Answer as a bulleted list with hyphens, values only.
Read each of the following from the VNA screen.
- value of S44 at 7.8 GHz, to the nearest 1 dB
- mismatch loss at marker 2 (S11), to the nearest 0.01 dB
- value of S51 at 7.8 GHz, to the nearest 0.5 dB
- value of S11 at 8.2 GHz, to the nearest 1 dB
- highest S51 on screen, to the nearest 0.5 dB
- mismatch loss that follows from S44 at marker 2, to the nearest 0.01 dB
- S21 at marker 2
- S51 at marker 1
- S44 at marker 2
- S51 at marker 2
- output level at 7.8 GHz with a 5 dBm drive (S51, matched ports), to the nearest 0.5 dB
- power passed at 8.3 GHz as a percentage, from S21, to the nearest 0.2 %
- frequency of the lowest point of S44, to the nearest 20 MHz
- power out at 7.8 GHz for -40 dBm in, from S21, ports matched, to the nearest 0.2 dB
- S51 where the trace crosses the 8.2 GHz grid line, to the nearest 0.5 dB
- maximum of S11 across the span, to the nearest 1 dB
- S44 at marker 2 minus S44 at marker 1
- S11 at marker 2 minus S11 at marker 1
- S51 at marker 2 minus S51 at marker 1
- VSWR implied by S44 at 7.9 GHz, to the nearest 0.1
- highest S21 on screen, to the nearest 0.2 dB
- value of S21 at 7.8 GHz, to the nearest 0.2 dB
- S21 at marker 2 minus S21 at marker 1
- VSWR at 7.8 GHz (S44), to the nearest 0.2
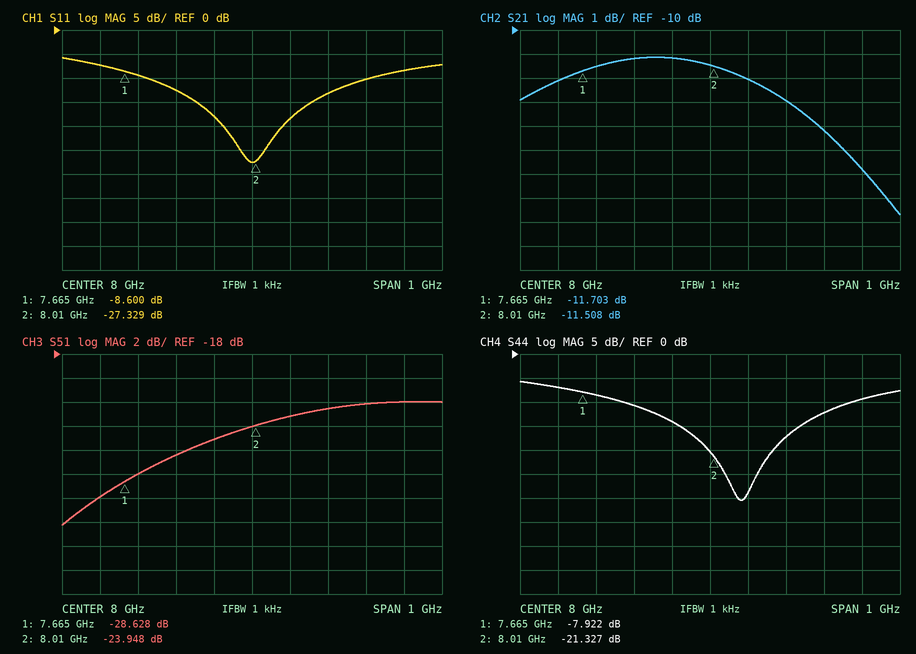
- -11 dB
- 0.01 dB
- -26.5 dB
- -13 dB
- -22.0 dB
- 0.03 dB
- -11.508 dB
- -28.628 dB
- -21.327 dB
- -23.948 dB
- -21.5 dBm
- 3.8 %
- 8.08 GHz
- -51.2 dBm
- -22.5 dB
- -6 dB
- -13.405 dB
- -18.729 dB
- 4.680 dB
- 1.5
- -11.2 dB
- -11.2 dB
- 0.195 dB
- 1.8
